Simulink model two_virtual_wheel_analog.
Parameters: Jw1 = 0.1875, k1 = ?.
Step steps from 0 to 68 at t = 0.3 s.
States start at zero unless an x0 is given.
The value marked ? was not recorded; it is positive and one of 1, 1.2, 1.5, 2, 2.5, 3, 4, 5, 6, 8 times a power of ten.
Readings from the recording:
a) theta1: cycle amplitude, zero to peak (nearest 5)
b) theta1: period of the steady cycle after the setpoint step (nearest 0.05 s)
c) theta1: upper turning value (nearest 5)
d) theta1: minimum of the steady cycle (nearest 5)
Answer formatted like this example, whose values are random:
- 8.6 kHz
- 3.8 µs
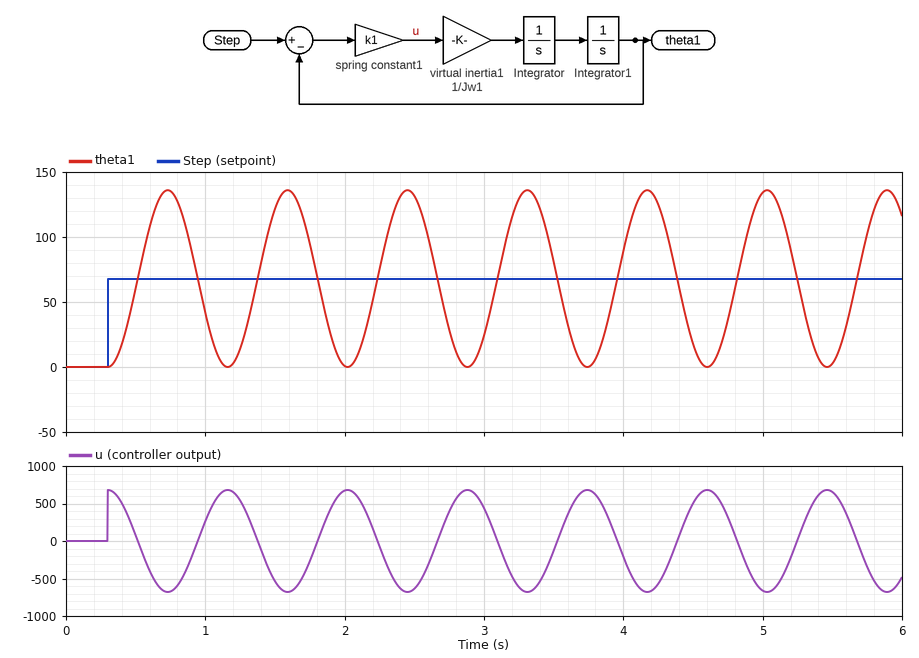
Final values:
- 70
- 0.85 s
- 135
- 0
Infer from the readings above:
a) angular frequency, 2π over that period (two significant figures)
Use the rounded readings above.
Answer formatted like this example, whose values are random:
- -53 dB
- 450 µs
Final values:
- 7.4 rad/s
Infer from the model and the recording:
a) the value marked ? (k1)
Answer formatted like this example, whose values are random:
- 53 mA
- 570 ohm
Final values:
- 10
